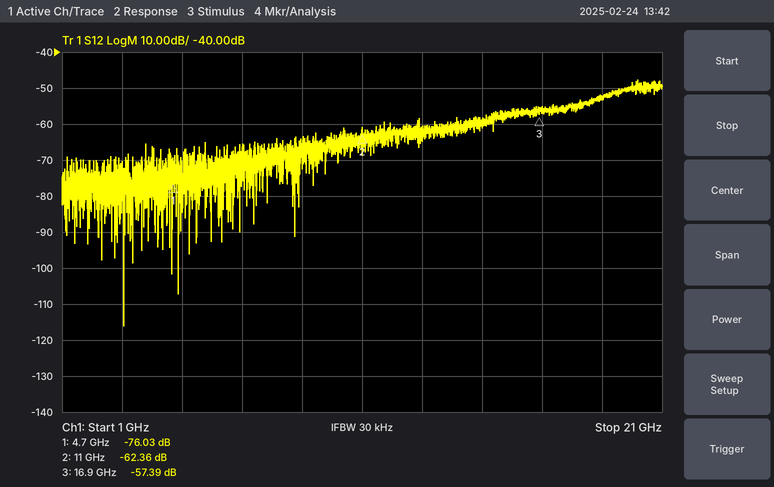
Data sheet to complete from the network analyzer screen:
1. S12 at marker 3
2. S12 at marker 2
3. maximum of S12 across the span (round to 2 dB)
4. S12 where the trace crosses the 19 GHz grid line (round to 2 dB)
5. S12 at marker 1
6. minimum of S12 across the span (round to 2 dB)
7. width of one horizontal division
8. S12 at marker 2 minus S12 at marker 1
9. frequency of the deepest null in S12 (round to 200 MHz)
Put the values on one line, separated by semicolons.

-57.39 dB; -62.36 dB; -48 dB; -52 dB; -76.03 dB; -116 dB; 2 GHz; 13.67 dB; 3.0 GHz
